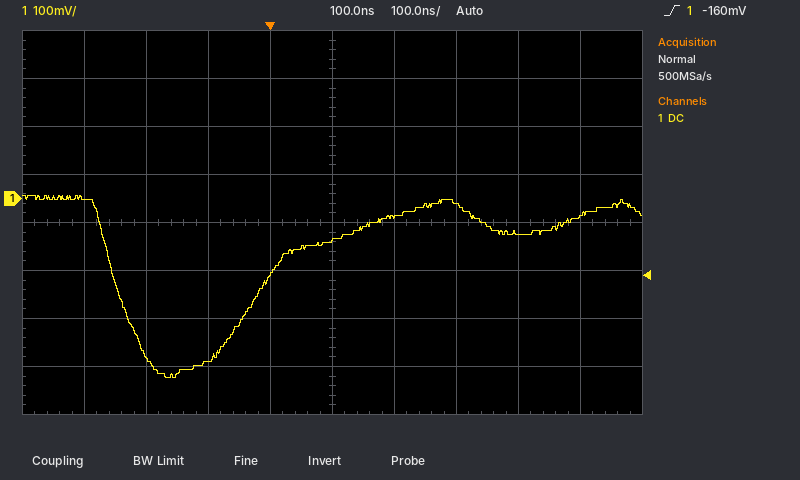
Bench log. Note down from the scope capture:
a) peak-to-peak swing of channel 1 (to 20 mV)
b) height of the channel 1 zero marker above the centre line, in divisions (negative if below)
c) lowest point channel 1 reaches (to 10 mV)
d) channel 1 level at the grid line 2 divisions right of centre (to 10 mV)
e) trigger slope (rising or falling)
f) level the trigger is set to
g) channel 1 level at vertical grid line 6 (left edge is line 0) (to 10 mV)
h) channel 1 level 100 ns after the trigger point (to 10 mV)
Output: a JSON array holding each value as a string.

["380 mV", "+0.5 div", "-370 mV", "-10 mV", "rising", "-160 mV", "-40 mV", "-90 mV"]
